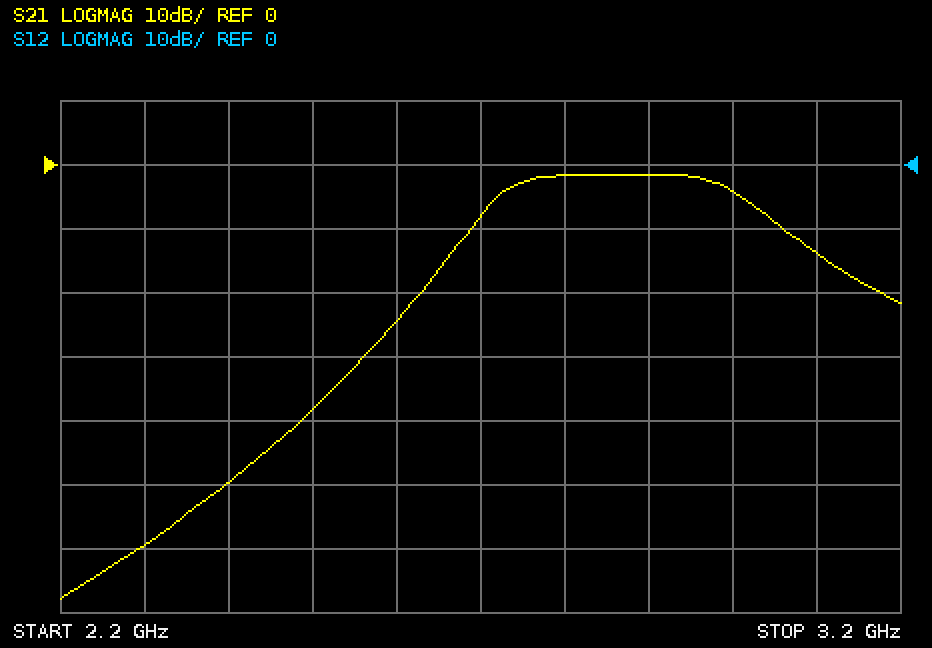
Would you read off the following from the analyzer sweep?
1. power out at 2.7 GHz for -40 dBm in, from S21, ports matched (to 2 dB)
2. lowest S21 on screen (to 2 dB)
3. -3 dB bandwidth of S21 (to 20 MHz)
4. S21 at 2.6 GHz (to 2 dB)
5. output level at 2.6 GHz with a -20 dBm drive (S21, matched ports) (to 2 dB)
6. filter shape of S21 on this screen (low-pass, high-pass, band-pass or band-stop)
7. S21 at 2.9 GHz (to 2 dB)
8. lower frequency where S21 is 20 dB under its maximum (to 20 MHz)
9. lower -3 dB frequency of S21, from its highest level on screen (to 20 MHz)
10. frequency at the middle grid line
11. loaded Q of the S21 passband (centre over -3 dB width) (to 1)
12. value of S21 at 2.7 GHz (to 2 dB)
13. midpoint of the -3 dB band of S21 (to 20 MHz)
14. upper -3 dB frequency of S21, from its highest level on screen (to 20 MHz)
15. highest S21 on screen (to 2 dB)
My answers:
-48 dBm
-68 dB
280 MHz
-24 dB
-44 dBm
band-pass
-2 dB
2.62 GHz
2.72 GHz
2.7 GHz
10
-8 dB
2.86 GHz
3.00 GHz
-2 dB
